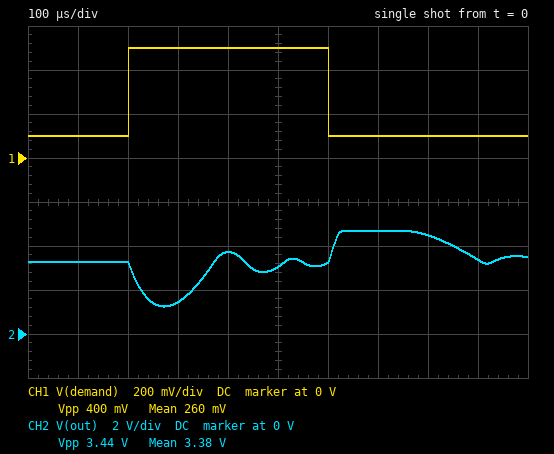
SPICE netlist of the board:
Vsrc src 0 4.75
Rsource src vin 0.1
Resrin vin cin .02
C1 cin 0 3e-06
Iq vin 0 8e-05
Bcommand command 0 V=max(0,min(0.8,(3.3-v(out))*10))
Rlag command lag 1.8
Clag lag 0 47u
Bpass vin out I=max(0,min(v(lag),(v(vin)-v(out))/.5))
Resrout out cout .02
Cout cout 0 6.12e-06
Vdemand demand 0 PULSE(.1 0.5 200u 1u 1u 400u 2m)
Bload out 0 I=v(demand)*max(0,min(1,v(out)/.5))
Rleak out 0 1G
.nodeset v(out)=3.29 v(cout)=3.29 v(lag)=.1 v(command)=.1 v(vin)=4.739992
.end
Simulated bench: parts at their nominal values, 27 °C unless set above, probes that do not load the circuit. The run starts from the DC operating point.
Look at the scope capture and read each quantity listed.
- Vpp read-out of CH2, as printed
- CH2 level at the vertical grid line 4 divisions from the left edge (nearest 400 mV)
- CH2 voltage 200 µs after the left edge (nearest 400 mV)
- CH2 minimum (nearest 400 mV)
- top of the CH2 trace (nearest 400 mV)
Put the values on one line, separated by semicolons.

3.44 V; 3.6 V; 3.2 V; 1.2 V; 4.8 V
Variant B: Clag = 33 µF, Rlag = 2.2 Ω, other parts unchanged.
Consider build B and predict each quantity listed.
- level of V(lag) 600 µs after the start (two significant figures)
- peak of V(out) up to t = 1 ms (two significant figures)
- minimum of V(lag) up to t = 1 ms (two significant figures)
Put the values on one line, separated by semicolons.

550 mV; 4.7 V; 13 mV
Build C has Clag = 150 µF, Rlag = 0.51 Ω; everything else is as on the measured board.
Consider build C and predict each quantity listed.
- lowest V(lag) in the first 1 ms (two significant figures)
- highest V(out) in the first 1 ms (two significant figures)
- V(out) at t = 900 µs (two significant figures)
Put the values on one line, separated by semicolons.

14 mV; 4.7 V; 3.3 V
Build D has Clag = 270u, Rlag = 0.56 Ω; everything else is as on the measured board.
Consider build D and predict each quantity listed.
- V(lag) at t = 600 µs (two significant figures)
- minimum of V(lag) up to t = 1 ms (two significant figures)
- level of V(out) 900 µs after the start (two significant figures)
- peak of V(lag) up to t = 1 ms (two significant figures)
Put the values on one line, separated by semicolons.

390 mV; 31 mV; 4.4 V; 690 mV
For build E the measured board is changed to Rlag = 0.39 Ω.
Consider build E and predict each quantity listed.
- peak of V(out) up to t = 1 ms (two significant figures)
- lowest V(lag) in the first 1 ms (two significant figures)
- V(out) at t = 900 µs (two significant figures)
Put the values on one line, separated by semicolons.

4.0 V; 4.0 mV; 3.3 V
